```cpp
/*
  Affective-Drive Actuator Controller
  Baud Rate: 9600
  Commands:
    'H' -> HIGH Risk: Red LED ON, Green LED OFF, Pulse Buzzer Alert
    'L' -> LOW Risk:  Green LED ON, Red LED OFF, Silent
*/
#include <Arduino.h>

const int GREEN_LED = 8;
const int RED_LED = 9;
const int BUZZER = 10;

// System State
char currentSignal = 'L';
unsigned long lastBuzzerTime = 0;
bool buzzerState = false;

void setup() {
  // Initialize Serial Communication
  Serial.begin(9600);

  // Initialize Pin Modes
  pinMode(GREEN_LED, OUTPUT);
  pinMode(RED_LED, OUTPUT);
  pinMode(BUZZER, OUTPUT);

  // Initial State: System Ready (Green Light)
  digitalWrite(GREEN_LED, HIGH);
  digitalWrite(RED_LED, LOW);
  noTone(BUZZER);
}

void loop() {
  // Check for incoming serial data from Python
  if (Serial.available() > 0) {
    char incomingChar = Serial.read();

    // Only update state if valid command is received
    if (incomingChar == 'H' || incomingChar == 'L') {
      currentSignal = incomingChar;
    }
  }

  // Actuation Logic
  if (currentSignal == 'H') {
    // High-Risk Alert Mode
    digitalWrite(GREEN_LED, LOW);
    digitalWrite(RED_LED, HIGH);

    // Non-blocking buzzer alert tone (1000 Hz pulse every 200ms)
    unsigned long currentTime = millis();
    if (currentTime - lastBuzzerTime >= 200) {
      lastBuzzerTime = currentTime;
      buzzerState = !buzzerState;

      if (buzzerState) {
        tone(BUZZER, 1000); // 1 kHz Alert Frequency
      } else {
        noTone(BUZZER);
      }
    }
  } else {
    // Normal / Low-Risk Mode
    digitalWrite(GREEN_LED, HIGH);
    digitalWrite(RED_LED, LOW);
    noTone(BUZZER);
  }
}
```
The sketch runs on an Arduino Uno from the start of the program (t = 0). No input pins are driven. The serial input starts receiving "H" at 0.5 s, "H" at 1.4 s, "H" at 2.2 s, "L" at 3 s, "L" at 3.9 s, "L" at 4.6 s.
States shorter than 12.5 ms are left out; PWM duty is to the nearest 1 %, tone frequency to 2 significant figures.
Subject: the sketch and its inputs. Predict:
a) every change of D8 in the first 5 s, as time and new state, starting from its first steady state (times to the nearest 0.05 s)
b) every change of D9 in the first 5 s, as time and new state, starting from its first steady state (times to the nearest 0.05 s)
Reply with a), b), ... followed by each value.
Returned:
a) 0 s high; 0.5 s low; 3 s high
b) 0 s low; 0.5 s high; 3 s low
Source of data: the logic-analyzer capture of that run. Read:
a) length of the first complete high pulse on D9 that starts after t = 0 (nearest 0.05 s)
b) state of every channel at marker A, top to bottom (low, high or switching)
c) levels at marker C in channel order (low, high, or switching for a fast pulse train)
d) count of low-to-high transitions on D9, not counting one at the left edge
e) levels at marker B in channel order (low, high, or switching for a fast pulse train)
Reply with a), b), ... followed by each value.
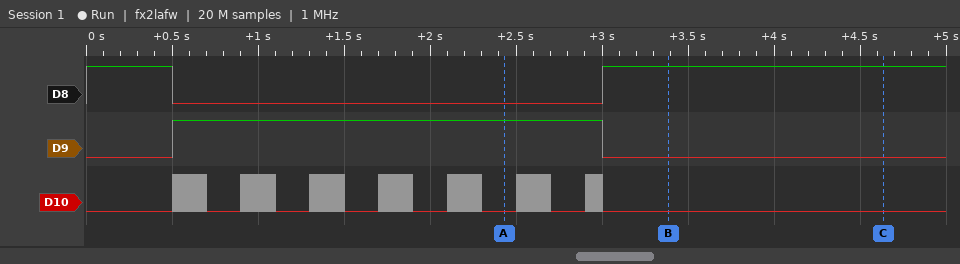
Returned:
a) 2.50 s
b) D8 low, D9 high, D10 low
c) D8 high, D9 low, D10 low
d) 1
e) D8 high, D9 low, D10 low
